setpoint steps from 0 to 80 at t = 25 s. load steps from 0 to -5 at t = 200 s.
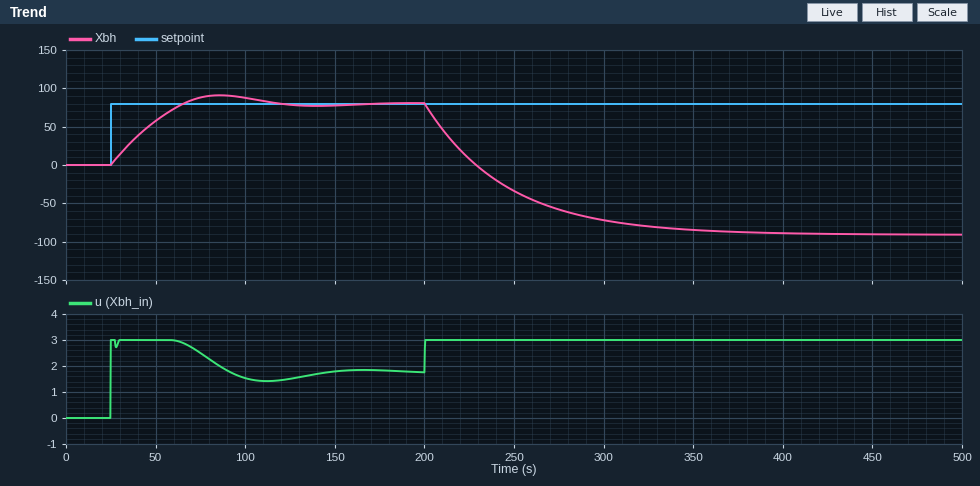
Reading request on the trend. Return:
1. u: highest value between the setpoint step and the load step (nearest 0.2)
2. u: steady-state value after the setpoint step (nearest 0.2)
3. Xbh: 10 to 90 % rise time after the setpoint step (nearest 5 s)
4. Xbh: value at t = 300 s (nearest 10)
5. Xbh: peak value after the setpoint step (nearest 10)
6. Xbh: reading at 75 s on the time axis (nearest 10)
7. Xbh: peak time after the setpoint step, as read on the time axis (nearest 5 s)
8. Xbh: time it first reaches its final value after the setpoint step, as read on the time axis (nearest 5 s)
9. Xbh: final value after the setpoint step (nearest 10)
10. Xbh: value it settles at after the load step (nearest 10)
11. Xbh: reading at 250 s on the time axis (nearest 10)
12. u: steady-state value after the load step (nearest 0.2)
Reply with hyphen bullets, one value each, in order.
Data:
- 3.0
- 1.8
- 30 s
- -70
- 90
- 90
- 85 s
- 65 s
- 80
- -90
- -30
- 3.0
